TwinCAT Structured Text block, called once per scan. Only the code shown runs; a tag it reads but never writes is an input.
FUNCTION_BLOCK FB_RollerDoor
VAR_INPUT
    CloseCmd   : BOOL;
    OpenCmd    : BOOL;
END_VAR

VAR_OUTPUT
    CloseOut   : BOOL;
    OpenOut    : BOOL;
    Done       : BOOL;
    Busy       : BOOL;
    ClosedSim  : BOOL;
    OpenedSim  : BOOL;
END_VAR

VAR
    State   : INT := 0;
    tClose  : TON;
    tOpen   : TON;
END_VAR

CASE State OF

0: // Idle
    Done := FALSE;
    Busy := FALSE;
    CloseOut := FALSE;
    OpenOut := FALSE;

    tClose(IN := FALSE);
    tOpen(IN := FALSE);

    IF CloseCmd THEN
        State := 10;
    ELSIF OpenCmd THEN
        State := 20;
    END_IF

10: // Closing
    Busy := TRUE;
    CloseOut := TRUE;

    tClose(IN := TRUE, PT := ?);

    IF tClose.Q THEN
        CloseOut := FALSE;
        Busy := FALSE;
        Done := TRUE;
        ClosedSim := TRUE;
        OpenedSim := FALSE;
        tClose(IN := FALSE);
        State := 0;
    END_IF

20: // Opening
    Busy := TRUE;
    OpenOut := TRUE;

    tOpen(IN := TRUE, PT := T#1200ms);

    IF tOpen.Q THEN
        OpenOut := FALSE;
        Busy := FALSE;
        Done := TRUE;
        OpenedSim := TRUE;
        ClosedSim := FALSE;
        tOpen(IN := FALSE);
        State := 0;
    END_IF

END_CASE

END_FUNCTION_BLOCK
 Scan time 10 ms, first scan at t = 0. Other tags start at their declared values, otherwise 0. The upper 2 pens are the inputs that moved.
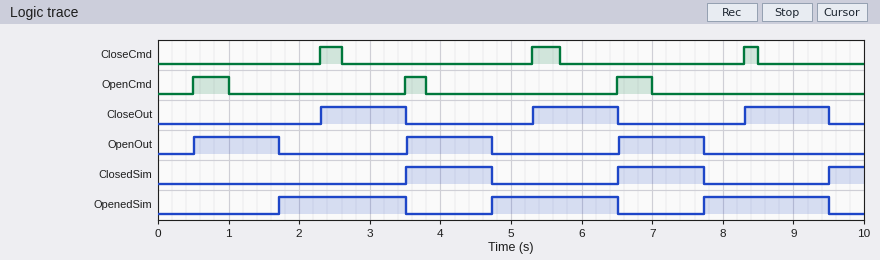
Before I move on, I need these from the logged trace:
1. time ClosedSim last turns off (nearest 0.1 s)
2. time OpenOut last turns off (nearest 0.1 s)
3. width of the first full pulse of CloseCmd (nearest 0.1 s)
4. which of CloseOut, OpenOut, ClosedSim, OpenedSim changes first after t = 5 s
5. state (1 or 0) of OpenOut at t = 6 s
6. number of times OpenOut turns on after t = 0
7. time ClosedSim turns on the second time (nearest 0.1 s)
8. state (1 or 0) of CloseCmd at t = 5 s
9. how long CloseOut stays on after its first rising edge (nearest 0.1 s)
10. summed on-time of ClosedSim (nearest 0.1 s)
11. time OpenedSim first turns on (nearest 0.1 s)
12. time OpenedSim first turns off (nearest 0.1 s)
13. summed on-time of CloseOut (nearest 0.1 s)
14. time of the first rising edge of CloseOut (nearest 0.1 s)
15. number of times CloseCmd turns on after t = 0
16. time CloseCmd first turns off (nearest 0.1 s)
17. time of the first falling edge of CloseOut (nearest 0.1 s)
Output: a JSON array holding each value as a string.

["7.7 s", "7.7 s", "0.3 s", "CloseOut", "0", "3", "6.5 s", "0", "1.2 s", "2.9 s", "1.7 s", "3.5 s", "3.6 s", "2.3 s", "3", "2.6 s", "3.5 s"]
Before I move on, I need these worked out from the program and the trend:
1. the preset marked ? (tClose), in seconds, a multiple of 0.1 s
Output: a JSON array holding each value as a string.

["1.2 s"]
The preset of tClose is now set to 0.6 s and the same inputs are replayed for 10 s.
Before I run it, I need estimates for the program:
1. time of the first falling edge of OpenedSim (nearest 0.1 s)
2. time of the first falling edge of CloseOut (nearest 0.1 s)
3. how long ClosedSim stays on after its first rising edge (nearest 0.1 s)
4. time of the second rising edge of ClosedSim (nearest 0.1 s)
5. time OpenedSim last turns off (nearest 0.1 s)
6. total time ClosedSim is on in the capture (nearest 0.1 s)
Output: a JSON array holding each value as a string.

["2.9 s", "2.9 s", "1.8 s", "5.9 s", "8.9 s", "4.7 s"]
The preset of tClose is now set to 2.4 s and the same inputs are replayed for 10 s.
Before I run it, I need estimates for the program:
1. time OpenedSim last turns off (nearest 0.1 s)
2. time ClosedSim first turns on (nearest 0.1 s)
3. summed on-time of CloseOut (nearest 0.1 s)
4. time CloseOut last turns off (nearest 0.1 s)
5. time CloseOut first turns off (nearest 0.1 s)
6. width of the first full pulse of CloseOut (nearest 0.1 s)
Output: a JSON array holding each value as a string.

["4.7 s", "4.7 s", "6.5 s", "7.7 s", "4.7 s", "2.4 s"]
